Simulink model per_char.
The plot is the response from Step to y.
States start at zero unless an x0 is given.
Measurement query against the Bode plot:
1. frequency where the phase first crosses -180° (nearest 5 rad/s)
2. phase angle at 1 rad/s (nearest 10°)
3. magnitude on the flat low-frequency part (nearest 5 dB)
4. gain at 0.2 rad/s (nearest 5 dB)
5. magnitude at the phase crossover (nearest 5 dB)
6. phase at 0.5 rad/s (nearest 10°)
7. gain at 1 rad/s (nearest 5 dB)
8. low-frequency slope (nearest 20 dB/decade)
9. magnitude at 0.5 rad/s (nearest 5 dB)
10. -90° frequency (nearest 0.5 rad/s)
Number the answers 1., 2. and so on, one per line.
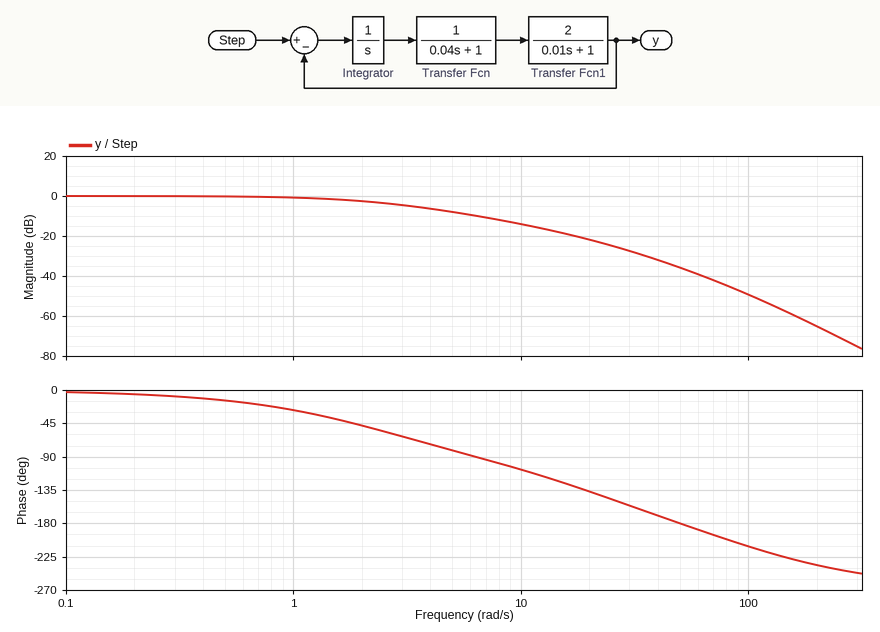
1. 50 rad/s
2. -30°
3. 0 dB
4. 0 dB
5. -35 dB
6. -10°
7. 0 dB
8. 0 dB/decade
9. 0 dB
10. 6.5 rad/s
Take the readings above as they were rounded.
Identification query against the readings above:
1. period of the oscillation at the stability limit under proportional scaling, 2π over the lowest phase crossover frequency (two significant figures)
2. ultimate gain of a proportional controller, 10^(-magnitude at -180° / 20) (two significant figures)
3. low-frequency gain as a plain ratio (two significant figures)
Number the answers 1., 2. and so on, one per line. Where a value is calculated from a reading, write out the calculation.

1. 2π / 50 = 0.13 s
2. 10^(35 / 20) = 56
3. 10^(0 / 20) = 1.0
